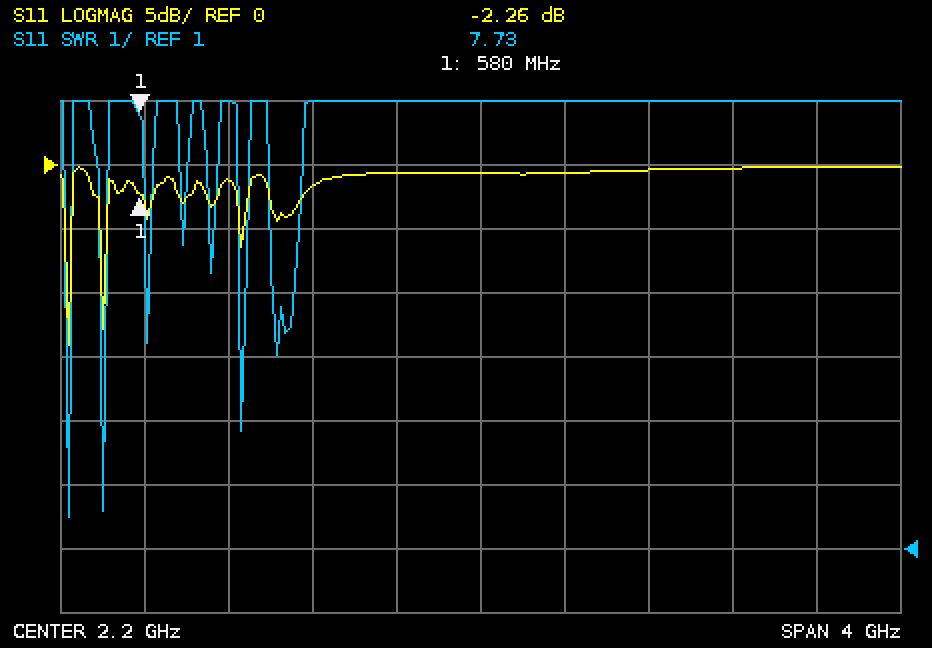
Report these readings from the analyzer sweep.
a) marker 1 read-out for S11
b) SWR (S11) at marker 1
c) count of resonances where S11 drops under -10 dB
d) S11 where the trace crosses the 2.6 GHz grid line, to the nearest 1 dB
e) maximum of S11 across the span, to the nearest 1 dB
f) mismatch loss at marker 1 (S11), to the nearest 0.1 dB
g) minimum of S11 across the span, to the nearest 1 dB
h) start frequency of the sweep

-2.26 dB
7.73
2
-1 dB
0 dB
3.9 dB
-14 dB
200 MHz
